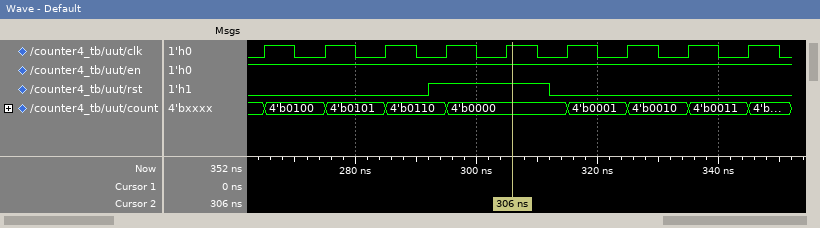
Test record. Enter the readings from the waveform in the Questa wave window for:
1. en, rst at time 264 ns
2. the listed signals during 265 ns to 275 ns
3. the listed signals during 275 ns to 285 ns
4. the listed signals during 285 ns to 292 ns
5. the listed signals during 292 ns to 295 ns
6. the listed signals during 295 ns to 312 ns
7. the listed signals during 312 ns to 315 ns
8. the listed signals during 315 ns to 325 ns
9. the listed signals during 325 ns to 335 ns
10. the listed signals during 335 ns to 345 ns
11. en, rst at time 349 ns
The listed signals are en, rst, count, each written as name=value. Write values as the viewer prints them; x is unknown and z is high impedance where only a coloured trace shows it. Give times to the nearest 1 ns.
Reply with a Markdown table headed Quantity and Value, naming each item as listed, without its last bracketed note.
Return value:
| Quantity | Value |
|---|---|
| en, rst at time 264 ns | en=1, rst=0 |
| the listed signals during 265 ns to 275 ns | en=1, rst=0, count=4'b0100 |
| the listed signals during 275 ns to 285 ns | en=1, rst=0, count=4'b0101 |
| the listed signals during 285 ns to 292 ns | en=1, rst=0, count=4'b0110 |
| the listed signals during 292 ns to 295 ns | en=1, rst=1, count=4'b0110 |
| the listed signals during 295 ns to 312 ns | en=1, rst=1, count=4'b0000 |
| the listed signals during 312 ns to 315 ns | en=1, rst=0, count=4'b0000 |
| the listed signals during 315 ns to 325 ns | en=1, rst=0, count=4'b0001 |
| the listed signals during 325 ns to 335 ns | en=1, rst=0, count=4'b0010 |
| the listed signals during 335 ns to 345 ns | en=1, rst=0, count=4'b0011 |
| en, rst at time 349 ns | en=1, rst=0 |
